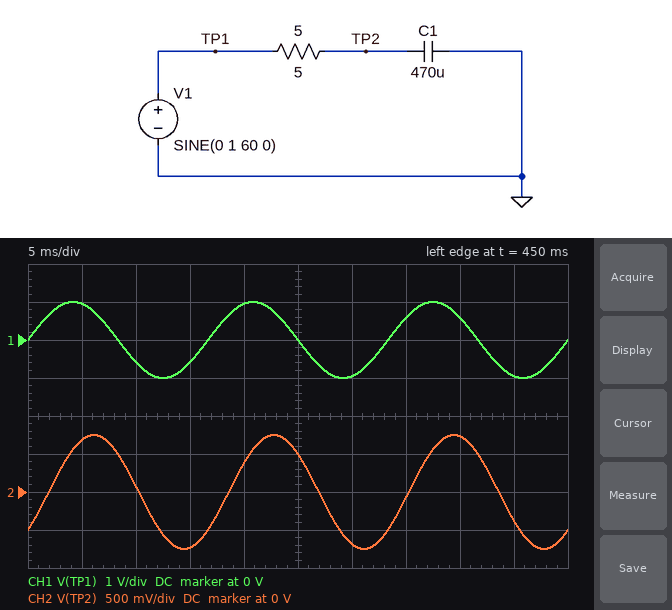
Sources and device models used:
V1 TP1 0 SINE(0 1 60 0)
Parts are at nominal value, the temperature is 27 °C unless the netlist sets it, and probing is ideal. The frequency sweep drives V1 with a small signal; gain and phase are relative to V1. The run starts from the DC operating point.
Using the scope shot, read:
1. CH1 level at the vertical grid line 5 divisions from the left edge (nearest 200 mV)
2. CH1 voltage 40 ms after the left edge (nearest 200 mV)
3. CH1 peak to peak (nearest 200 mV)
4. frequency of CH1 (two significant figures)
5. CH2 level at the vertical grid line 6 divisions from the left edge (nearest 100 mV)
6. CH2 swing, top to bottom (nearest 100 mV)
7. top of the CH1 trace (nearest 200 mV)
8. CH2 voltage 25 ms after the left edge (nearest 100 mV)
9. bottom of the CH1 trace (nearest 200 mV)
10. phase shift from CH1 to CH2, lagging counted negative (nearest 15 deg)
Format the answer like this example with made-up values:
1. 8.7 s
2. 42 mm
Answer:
1. 0 V
2. 600 mV
3. 2.0 V
4. 60 Hz
5. -700 mV
6. 1.5 V
7. 1.0 V
8. 500 mV
9. -1.0 V
10. -45 deg
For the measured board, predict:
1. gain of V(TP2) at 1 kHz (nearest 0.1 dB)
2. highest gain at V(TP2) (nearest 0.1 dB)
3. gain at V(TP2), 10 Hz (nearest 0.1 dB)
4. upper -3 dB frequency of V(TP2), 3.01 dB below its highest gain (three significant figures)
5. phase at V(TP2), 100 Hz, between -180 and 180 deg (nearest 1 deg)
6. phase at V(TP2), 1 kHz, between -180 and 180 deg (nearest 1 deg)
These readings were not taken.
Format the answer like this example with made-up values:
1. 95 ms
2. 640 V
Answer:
1. -23.4 dB
2. 0 dB
3. -0.1 dB
4. 67.7 Hz
5. -56 deg
6. -86 deg
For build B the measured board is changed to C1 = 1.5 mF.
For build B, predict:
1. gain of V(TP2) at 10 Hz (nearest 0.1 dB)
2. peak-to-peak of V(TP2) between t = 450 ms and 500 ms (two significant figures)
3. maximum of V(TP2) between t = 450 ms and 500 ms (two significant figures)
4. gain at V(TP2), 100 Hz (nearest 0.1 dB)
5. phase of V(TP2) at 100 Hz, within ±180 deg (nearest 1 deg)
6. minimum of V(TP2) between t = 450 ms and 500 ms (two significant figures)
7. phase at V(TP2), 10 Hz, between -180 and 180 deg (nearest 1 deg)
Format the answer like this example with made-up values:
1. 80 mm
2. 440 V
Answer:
1. -0.9 dB
2. 670 mV
3. 330 mV
4. -13.7 dB
5. -78 deg
6. -330 mV
7. -25 deg
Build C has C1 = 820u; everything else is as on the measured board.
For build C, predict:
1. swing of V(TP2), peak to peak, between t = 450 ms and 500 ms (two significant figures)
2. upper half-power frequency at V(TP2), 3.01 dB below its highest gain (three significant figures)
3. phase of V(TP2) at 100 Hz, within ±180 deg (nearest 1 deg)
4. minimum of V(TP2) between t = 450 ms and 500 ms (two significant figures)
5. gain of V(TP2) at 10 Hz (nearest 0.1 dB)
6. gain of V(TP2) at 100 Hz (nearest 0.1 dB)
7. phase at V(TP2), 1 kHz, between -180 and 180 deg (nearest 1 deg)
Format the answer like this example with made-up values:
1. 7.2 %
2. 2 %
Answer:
1. 1.1 V
2. 38.8 Hz
3. -69 deg
4. -540 mV
5. -0.3 dB
6. -8.8 dB
7. -88 deg
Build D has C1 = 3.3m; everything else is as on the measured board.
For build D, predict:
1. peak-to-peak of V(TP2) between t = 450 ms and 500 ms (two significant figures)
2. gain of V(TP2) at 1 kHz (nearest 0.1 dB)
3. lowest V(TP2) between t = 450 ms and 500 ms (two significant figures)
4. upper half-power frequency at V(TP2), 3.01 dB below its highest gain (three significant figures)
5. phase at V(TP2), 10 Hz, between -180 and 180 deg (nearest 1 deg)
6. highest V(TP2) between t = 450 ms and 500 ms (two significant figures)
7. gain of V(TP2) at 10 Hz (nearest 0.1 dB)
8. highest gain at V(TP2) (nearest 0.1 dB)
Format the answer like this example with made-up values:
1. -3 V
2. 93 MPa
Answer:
1. 320 mV
2. -40.3 dB
3. -160 mV
4. 9.65 Hz
5. -46 deg
6. 160 mV
7. -3.2 dB
8. 0 dB
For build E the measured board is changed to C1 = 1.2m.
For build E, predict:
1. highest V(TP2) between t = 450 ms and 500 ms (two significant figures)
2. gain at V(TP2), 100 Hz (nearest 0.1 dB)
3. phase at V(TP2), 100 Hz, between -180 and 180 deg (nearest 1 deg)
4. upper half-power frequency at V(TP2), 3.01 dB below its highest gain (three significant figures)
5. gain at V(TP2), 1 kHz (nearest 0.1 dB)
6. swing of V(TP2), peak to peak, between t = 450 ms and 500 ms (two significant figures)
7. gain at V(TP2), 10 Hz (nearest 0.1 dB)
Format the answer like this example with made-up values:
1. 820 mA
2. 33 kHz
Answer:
1. 400 mV
2. -11.8 dB
3. -75 deg
4. 26.5 Hz
5. -31.5 dB
6. 810 mV
7. -0.6 dB
